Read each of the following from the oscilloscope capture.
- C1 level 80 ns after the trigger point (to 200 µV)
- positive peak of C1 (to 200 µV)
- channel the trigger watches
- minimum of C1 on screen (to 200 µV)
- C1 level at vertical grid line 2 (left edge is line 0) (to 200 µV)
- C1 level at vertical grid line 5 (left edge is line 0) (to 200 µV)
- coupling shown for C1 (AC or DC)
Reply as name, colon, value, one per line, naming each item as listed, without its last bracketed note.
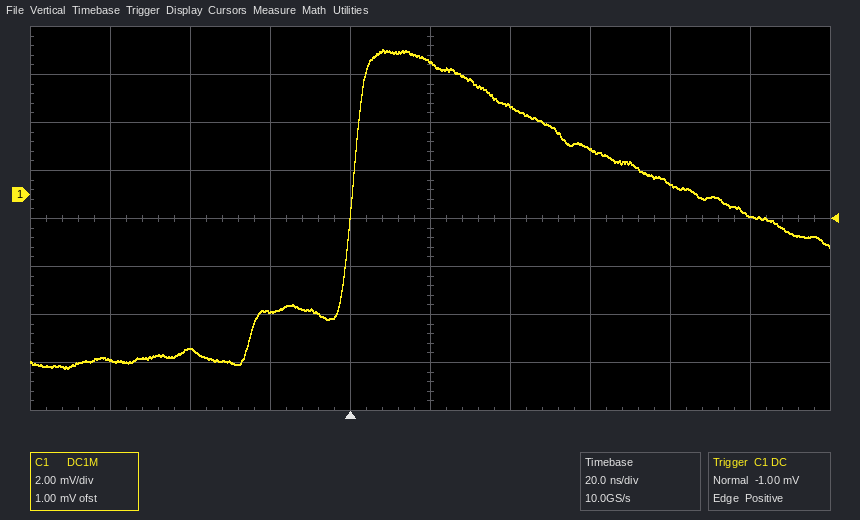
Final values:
C1 level 80 ns after the trigger point: 400 µV
positive peak of C1: 6.0 mV
channel the trigger watches: C1
minimum of C1 on screen: -7.2 mV
C1 level at vertical grid line 2 (left edge is line 0): -6.4 mV
C1 level at vertical grid line 5 (left edge is line 0): 5.6 mV
coupling shown for C1: DC
